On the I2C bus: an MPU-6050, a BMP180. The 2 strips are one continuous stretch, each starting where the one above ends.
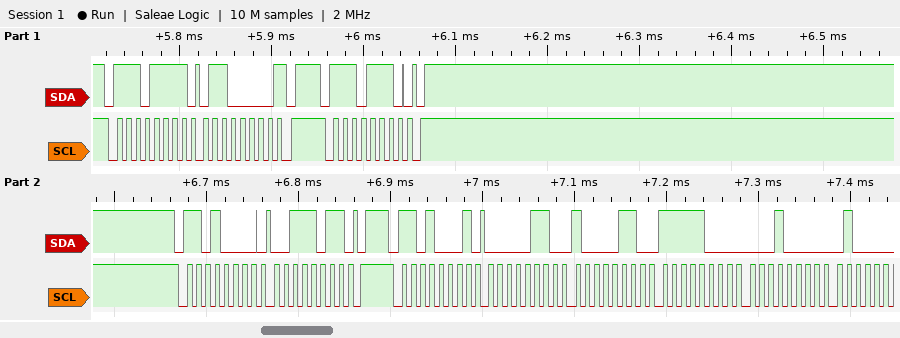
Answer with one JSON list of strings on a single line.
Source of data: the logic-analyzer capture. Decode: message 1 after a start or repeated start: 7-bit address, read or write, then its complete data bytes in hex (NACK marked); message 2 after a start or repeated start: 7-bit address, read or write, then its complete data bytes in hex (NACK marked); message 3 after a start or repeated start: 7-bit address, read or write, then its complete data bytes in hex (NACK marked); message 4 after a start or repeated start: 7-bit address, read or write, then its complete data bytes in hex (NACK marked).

["0x77 read: 60 NACK", "0x77 write", "0x68 write: 3B", "0x68 read: 06 86 F8 10"]
